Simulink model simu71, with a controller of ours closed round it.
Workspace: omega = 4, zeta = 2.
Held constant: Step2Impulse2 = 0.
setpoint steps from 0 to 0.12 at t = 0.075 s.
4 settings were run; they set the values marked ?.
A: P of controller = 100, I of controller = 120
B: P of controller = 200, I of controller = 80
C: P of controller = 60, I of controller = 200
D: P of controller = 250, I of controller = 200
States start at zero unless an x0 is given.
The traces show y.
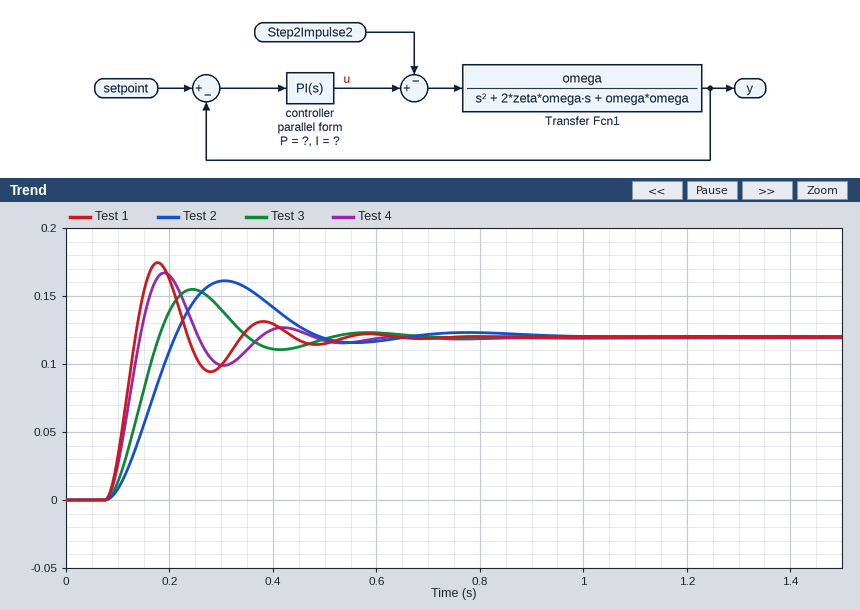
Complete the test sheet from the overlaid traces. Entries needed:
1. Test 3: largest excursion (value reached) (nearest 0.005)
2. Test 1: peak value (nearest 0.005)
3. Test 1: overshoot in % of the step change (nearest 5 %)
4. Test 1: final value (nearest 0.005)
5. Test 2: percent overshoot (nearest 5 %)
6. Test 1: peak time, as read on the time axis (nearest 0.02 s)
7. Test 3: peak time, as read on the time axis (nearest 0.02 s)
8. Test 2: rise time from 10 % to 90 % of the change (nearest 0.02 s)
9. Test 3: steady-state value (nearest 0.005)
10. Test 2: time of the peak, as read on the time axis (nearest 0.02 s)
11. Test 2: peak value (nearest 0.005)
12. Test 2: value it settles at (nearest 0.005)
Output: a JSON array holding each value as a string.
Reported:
["0.155", "0.175", "45 %", "0.120", "35 %", "0.18 s", "0.24 s", "0.10 s", "0.120", "0.30 s", "0.160", "0.120"]
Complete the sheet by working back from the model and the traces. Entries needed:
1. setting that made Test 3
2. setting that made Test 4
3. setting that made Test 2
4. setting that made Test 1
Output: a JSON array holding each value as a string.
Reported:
["A", "B", "C", "D"]
